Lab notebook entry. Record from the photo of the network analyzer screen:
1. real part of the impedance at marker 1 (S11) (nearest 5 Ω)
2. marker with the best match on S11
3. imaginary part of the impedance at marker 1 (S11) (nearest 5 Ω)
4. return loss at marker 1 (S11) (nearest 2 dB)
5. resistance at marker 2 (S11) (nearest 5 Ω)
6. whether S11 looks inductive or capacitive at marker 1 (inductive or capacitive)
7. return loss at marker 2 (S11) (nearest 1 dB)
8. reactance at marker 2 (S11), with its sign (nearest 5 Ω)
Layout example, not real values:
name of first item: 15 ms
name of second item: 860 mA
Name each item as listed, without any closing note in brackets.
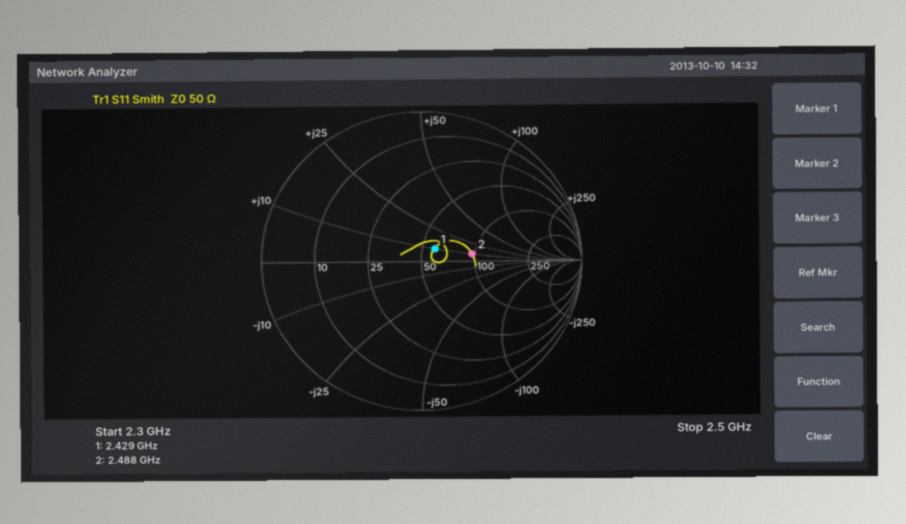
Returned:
real part of the impedance at marker 1 (S11): 60 Ω
marker with the best match on S11: marker 1
imaginary part of the impedance at marker 1 (S11): +10 Ω
return loss at marker 1 (S11): 18 dB
resistance at marker 2 (S11): 95 Ω
whether S11 looks inductive or capacitive at marker 1: inductive
return loss at marker 2 (S11): 10 dB
reactance at marker 2 (S11), with its sign: +10 Ω
